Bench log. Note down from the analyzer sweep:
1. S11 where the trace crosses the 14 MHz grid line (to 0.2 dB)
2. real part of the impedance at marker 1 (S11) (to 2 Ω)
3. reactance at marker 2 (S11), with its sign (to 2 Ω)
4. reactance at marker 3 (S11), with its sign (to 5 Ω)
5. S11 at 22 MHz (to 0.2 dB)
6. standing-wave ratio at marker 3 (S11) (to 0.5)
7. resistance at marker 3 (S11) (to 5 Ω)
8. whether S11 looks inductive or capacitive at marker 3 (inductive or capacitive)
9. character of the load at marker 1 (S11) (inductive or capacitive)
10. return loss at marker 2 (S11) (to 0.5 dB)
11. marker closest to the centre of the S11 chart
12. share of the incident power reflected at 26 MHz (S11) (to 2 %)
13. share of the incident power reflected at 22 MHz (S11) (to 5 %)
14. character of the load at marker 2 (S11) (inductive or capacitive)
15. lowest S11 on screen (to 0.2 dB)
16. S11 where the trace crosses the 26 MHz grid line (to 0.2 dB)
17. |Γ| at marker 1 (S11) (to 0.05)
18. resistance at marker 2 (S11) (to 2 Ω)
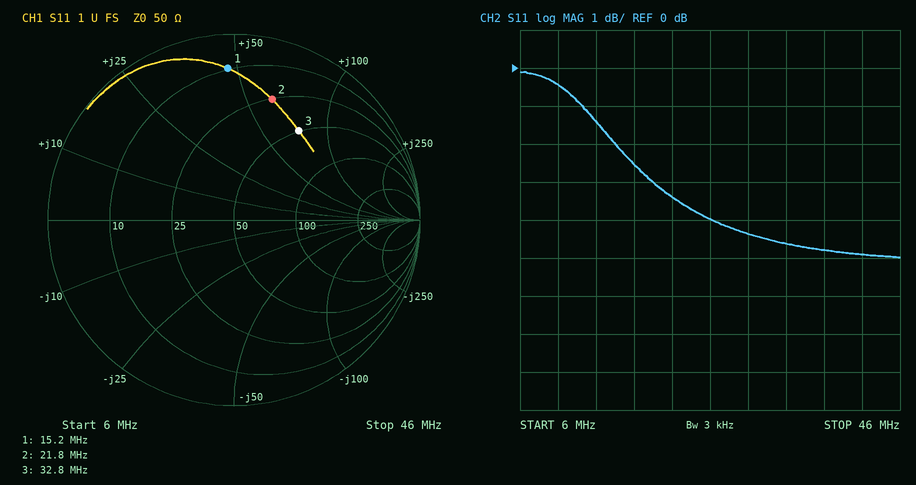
-1.4 dB
10 Ω
+62 Ω
+75 Ω
-3.4 dB
4.0
50 Ω
inductive
inductive
3.5 dB
marker 3
40 %
45 %
inductive
-5.0 dB
-4.0 dB
0.80
26 Ω
